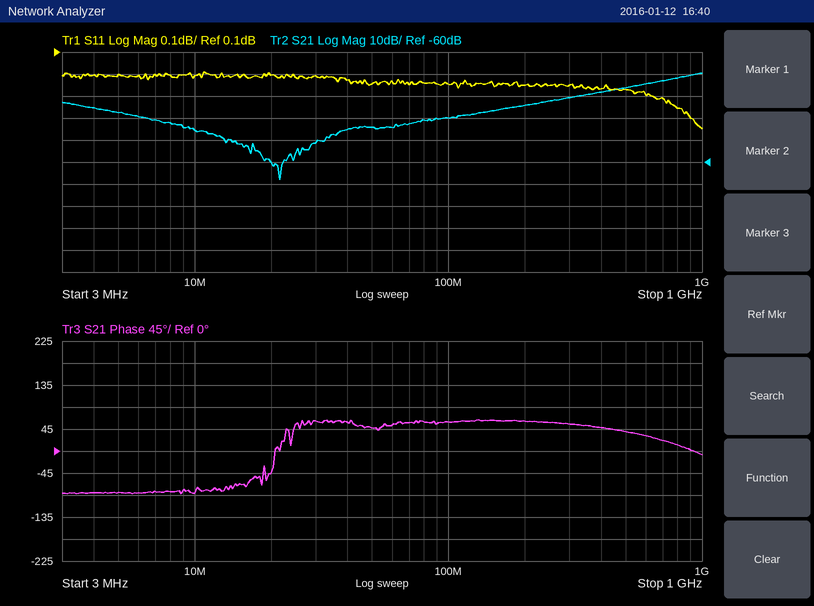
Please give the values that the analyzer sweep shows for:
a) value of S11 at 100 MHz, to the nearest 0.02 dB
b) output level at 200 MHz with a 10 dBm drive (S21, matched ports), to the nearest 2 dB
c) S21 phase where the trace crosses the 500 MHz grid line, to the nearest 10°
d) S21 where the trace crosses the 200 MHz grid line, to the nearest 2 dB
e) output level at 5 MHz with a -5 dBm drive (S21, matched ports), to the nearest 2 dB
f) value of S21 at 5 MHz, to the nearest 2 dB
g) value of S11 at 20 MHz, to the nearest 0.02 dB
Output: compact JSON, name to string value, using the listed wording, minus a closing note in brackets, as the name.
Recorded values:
{"value of S11 at 100 MHz, to the nearest 0.02 dB": "-0.04 dB", "output level at 200 MHz with a 10 dBm drive (S21, matched ports), to the nearest 2 dB": "-24 dBm", "S21 phase where the trace crosses the 500 MHz grid line, to the nearest 10°": "40°", "S21 where the trace crosses the 200 MHz grid line, to the nearest 2 dB": "-34 dB", "output level at 5 MHz with a -5 dBm drive (S21, matched ports), to the nearest 2 dB": "-42 dBm", "value of S21 at 5 MHz, to the nearest 2 dB": "-38 dB", "value of S11 at 20 MHz, to the nearest 0.02 dB": "0.00 dB"}
